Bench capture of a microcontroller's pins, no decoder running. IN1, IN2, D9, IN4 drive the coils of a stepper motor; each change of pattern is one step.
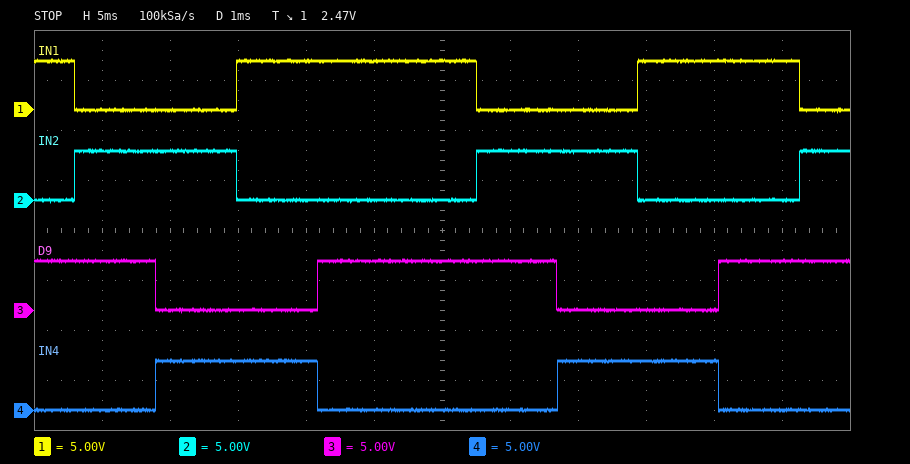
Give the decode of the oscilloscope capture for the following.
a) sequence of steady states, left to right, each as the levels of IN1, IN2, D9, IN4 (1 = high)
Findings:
1010 0110 0101 1001 1010 0110 0101 1001 1010 0110
